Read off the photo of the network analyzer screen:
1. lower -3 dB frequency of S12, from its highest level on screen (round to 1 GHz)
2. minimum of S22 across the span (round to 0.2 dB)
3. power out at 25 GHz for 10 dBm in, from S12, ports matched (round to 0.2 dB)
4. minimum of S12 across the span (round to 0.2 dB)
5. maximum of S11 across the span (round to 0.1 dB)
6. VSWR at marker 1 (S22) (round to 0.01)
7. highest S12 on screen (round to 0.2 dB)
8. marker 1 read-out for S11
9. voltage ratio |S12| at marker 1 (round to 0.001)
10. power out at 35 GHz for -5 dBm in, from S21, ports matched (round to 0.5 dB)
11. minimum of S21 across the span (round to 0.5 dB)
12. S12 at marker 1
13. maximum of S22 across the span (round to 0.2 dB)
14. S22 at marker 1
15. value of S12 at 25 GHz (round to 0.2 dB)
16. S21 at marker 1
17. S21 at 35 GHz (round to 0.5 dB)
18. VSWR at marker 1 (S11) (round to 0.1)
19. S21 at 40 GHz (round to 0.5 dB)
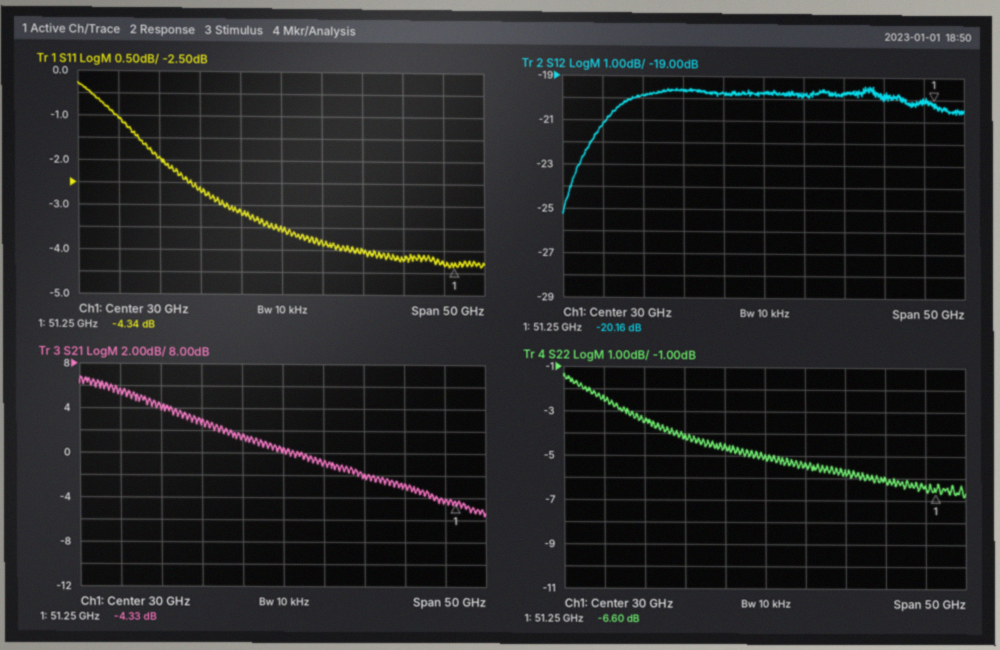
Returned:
8 GHz
-6.8 dB
-9.8 dBm
-25.2 dB
-0.3 dB
2.76
-19.4 dB
-4.34 dB
0.098
-6.0 dBm
-5.5 dB
-20.16 dB
-1.4 dB
-6.60 dB
-19.8 dB
-4.33 dB
-1.0 dB
4.1
-2.0 dB
